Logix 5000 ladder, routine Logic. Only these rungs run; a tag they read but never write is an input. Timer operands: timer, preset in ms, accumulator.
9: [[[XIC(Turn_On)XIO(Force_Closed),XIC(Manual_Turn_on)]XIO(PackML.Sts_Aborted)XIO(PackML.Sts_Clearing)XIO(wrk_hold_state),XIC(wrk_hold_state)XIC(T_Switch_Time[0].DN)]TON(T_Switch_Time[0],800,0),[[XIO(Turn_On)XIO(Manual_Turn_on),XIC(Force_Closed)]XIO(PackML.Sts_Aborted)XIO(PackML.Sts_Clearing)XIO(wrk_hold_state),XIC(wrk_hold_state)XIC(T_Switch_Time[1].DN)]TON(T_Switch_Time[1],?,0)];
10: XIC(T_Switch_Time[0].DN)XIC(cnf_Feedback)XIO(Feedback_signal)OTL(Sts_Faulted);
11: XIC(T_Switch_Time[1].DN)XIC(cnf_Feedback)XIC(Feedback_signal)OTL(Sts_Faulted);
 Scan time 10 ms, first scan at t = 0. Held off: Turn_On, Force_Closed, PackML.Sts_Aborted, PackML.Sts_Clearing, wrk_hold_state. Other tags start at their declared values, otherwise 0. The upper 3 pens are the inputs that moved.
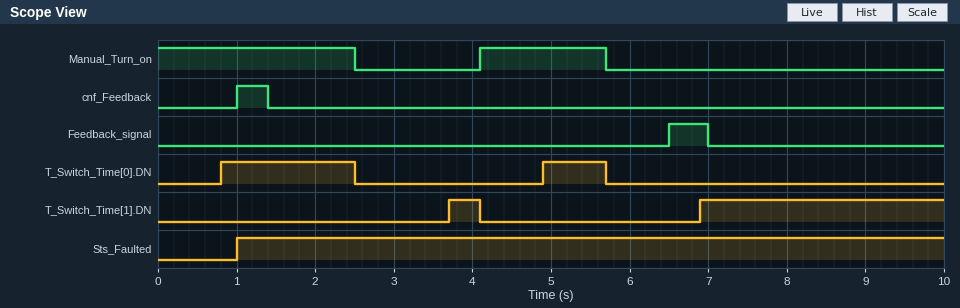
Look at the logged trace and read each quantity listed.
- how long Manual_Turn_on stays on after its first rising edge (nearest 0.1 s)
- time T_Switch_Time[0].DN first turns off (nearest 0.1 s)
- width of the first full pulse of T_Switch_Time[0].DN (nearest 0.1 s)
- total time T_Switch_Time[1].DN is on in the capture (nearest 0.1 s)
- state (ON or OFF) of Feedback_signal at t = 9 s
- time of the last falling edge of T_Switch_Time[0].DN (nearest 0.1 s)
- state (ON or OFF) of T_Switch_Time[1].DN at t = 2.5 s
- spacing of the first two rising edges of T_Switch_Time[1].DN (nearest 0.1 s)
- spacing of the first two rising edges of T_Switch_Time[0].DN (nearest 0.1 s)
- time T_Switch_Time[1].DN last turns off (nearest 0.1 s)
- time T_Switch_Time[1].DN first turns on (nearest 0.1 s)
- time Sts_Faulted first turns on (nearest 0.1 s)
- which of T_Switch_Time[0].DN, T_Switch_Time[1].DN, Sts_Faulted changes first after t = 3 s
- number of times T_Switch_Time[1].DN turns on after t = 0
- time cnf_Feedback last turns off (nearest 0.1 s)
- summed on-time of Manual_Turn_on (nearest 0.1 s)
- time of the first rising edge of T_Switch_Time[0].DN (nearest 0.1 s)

1.6 s
2.5 s
1.7 s
3.5 s
OFF
5.7 s
OFF
3.2 s
4.1 s
4.1 s
3.7 s
1.0 s
T_Switch_Time[1].DN
2
1.4 s
4.1 s
0.8 s
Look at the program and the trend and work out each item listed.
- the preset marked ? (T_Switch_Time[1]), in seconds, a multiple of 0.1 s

1.2 s
